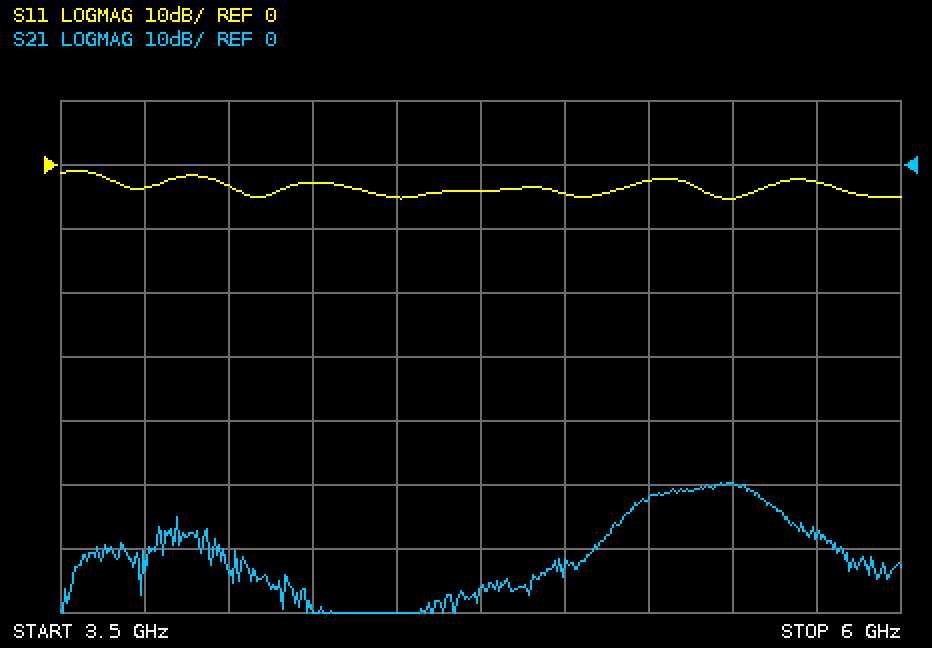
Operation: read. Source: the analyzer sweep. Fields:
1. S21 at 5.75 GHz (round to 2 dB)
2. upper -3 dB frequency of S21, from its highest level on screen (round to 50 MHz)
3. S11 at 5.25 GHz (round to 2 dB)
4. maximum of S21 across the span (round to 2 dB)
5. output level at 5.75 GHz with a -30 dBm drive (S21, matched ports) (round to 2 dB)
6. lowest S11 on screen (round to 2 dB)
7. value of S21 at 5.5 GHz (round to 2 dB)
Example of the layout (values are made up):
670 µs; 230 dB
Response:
-58 dB; 5.60 GHz; -2 dB; -50 dB; -88 dBm; -6 dB; -50 dB
